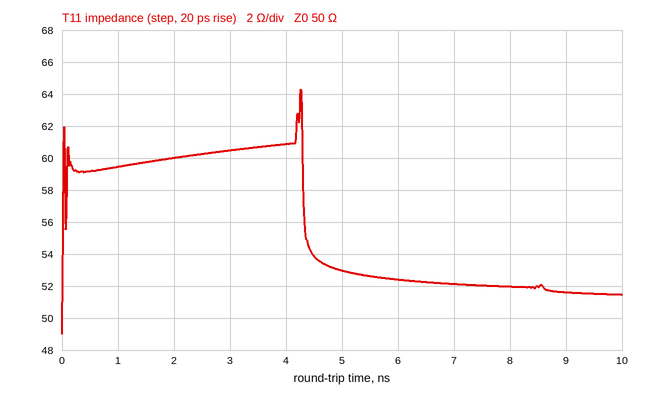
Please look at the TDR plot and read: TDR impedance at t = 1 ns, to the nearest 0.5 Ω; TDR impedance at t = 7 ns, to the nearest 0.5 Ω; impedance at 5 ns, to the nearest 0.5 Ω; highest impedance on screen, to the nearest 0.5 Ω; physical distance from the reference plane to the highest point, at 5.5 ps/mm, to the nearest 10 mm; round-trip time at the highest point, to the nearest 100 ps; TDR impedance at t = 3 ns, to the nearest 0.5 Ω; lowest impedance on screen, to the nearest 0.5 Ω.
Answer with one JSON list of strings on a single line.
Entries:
["59.5 Ω", "52.0 Ω", "53.0 Ω", "64.5 Ω", "390 mm", "4.3 ns", "60.5 Ω", "49.0 Ω"]
